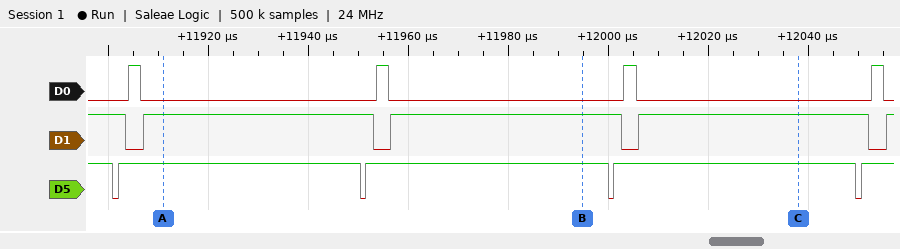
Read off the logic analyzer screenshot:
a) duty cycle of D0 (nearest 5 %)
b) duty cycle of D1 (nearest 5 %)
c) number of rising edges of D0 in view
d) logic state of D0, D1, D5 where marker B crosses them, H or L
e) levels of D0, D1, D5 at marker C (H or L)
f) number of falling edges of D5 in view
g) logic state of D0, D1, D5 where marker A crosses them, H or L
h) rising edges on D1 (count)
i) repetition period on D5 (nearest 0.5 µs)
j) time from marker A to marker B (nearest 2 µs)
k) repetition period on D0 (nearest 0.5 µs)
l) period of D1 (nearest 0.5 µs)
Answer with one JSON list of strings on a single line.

["5 %", "95 %", "4", "D0=L, D1=H, D5=H", "D0=L, D1=H, D5=H", "4", "D0=L, D1=H, D5=H", "4", "49.5 µs", "84 µs", "49.5 µs", "49.5 µs"]
